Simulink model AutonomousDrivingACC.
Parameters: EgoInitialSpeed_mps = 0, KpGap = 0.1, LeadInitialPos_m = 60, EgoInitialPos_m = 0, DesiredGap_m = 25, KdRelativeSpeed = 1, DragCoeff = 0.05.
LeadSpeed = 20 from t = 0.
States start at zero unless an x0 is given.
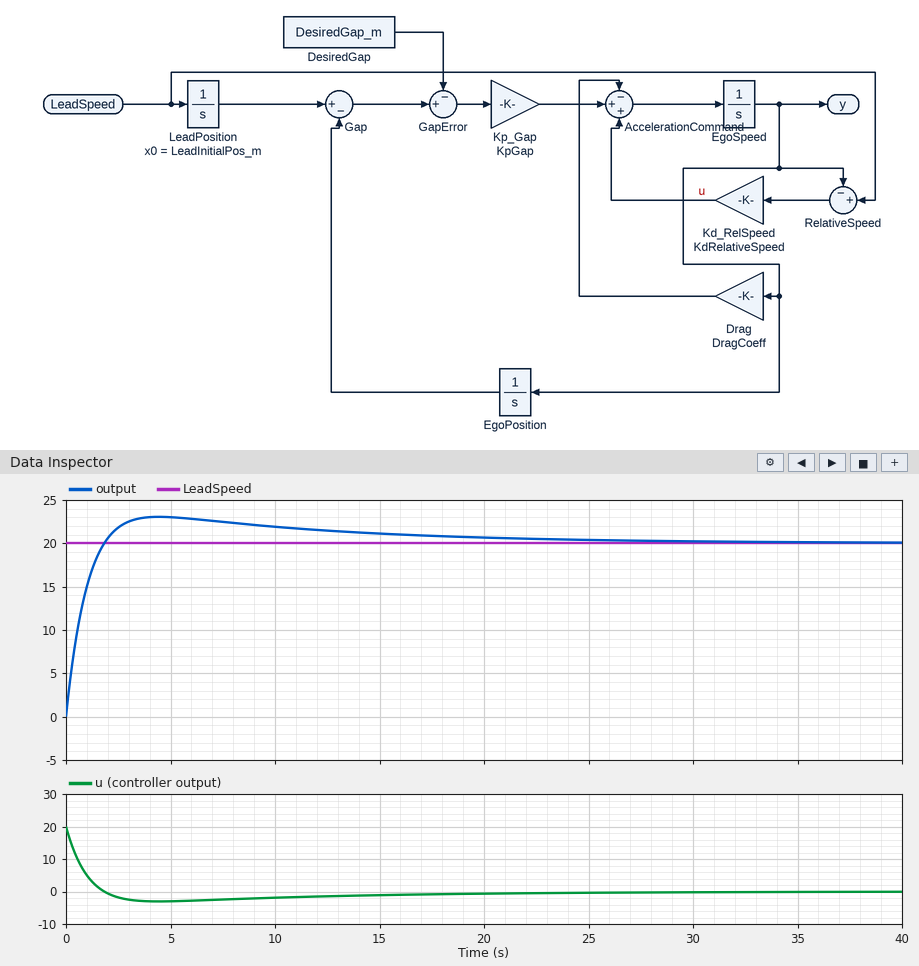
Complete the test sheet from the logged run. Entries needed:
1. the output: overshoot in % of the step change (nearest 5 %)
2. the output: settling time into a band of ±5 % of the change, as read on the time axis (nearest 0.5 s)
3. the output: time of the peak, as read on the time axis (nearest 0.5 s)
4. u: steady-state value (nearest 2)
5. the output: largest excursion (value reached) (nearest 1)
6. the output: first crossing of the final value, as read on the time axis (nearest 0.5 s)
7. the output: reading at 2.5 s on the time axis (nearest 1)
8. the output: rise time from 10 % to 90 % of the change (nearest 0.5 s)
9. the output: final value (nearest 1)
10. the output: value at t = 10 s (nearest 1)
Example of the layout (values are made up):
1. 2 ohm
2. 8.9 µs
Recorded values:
1. 15 %
2. 16.0 s
3. 4.5 s
4. 0
5. 23
6. 2.0 s
7. 22
8. 1.5 s
9. 20
10. 22
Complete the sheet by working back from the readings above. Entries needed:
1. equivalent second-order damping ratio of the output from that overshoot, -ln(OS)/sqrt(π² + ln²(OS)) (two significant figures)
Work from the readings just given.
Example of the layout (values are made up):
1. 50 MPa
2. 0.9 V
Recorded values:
1. 0.52
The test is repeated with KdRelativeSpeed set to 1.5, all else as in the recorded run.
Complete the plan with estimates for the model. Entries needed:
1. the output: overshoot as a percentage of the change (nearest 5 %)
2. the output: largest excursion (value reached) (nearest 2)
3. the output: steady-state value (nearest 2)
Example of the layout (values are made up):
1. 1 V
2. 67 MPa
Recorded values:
1. 10 %
2. 22
3. 20
